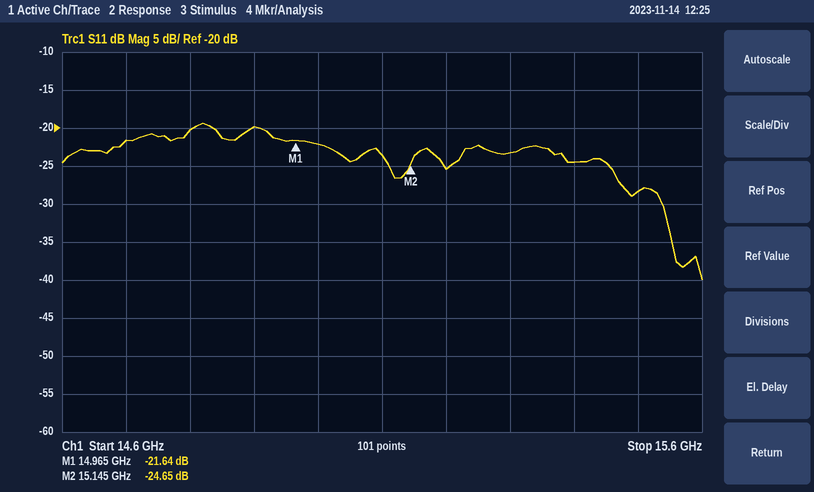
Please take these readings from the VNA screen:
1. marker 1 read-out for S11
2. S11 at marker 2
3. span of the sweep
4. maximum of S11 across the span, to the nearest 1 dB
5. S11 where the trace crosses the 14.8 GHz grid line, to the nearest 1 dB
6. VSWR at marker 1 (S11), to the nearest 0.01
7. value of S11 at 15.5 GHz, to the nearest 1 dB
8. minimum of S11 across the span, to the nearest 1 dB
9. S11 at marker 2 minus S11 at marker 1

-21.64 dB
-24.65 dB
1 GHz
-19 dB
-20 dB
1.18
-28 dB
-40 dB
-3.01 dB
